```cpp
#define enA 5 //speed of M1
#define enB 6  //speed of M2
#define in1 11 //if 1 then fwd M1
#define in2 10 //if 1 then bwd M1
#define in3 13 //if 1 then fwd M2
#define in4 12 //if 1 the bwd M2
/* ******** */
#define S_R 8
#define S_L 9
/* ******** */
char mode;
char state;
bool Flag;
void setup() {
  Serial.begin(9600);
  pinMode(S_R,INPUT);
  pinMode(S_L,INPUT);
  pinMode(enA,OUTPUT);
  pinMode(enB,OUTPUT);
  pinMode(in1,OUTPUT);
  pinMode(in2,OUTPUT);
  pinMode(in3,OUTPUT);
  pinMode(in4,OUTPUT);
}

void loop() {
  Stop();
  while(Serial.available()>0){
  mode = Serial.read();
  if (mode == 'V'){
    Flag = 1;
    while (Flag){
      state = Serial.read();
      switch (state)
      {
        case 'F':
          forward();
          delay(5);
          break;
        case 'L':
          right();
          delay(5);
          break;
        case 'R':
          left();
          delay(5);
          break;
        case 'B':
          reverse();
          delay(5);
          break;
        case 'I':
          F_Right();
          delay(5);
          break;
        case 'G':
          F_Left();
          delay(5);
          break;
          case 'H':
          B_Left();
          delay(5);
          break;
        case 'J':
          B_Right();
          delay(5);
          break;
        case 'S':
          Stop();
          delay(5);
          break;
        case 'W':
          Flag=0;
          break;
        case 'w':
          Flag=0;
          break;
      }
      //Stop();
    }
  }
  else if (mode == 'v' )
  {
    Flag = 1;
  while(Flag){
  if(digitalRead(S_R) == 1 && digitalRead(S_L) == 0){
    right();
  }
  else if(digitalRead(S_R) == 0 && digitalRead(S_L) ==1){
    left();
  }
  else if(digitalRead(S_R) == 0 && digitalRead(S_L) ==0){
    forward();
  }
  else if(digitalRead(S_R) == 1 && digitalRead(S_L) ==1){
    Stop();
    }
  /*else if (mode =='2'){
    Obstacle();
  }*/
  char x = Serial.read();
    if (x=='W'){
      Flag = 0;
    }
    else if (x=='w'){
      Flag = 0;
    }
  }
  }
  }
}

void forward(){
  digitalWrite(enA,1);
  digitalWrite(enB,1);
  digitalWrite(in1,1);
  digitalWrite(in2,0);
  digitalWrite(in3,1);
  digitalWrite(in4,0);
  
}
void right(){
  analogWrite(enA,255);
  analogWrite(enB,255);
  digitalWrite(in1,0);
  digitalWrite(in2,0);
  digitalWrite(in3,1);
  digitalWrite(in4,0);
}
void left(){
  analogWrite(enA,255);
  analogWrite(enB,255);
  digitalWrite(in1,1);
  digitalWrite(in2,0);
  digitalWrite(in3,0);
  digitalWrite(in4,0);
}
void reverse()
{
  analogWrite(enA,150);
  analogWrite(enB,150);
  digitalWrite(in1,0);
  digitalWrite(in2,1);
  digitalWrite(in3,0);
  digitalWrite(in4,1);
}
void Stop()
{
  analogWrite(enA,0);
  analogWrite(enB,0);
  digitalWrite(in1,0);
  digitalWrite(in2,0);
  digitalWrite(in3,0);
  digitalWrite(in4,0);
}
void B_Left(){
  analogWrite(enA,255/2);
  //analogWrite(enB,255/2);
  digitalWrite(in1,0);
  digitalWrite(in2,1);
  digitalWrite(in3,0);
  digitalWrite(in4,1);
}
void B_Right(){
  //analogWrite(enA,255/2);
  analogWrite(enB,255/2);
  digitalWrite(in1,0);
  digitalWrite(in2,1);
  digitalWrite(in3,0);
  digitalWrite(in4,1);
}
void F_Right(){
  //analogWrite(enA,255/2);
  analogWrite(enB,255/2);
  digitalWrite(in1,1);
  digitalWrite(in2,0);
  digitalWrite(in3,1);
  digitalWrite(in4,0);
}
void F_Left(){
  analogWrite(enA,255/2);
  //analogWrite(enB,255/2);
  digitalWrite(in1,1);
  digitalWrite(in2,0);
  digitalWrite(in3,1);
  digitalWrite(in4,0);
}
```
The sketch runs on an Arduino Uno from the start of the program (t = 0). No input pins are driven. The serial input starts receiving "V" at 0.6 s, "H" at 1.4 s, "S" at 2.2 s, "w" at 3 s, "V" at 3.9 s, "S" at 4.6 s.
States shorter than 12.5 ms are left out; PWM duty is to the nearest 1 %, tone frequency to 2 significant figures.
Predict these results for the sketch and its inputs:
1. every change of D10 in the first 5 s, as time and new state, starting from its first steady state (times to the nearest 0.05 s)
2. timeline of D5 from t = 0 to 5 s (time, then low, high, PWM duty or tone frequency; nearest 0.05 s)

0 s low; 1.4 s high; 2.2 s low
0 s low; 1.4 s PWM 50 %; 2.2 s low
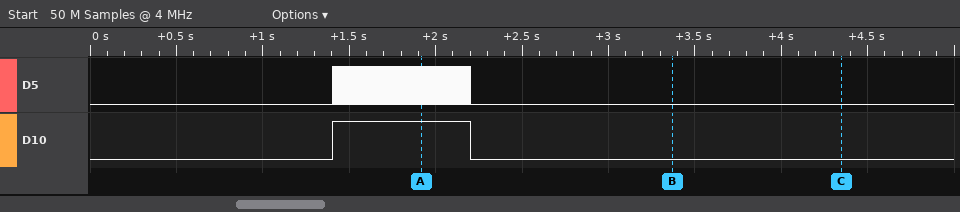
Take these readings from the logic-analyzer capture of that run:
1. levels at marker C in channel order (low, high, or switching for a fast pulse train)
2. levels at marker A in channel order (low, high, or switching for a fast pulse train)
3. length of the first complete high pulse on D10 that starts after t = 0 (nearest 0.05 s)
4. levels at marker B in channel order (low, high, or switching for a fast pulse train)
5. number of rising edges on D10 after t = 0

D5 low, D10 low
D5 switching, D10 high
0.80 s
D5 low, D10 low
1
